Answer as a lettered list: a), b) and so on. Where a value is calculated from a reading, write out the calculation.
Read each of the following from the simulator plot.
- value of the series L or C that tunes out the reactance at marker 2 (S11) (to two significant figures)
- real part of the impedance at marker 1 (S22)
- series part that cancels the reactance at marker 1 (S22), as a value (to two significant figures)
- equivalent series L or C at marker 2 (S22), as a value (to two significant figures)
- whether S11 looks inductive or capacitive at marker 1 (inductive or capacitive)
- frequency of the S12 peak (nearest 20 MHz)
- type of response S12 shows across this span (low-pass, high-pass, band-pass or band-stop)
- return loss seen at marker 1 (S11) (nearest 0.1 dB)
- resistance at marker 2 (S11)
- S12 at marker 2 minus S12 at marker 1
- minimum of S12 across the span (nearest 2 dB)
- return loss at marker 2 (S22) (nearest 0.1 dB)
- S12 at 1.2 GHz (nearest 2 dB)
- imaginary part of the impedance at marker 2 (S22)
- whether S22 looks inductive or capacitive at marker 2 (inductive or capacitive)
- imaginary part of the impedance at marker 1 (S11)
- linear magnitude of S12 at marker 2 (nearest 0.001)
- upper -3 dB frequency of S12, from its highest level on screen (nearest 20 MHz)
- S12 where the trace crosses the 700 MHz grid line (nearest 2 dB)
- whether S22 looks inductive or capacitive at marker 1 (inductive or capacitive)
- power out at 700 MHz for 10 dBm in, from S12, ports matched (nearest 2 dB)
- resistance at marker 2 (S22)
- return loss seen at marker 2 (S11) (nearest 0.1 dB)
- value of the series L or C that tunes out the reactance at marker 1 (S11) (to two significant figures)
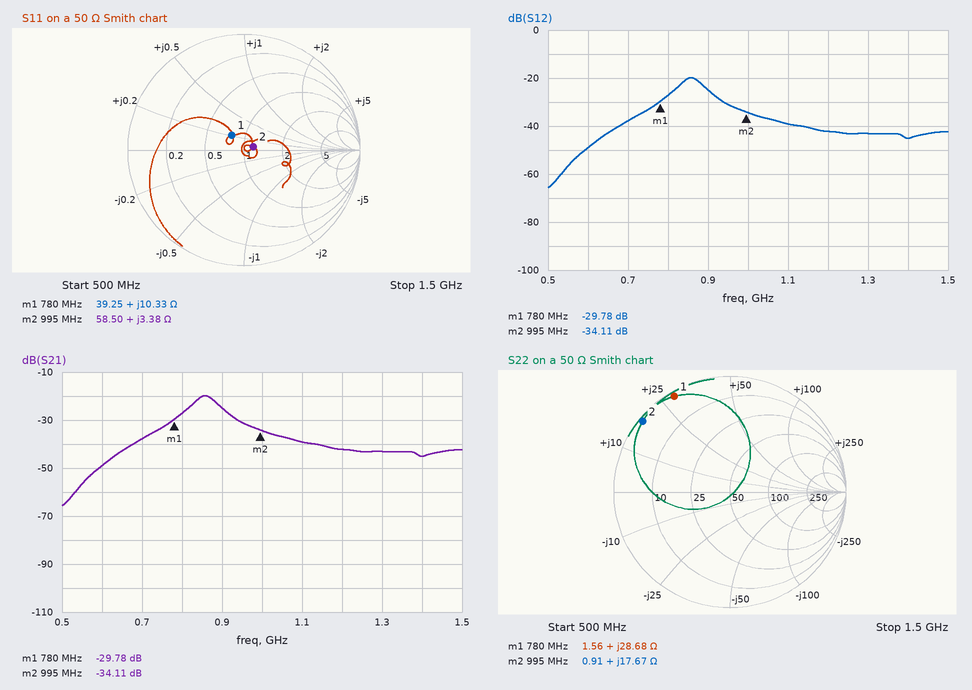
a) C = 1/(2π × 995 MHz × 3.38 Ω) ≈ 47 pF
b) 1.56 Ω
c) C = 1/(2π × 780 MHz × 28.68 Ω) ≈ 7.1 pF
d) L = 17.67 Ω/(2π × 995 MHz) ≈ 2.8 nH
e) inductive
f) 860 MHz
g) band-pass
h) 15.6 dB
i) 58.50 Ω
j) -34.11 − (-29.78) = -4.33 dB
k) -66 dB
l) 0.3 dB
m) -42 dB
n) +17.67 Ω
o) inductive
p) +10.33 Ω
q) 10^(-34.11/20) ≈ 0.020
r) 880 MHz
s) -38 dB
t) inductive
u) 10 dBm + (-38 dB) = -28 dBm
v) 0.91 Ω
w) 21.5 dB
x) C = 1/(2π × 780 MHz × 10.33 Ω) ≈ 20 pF
